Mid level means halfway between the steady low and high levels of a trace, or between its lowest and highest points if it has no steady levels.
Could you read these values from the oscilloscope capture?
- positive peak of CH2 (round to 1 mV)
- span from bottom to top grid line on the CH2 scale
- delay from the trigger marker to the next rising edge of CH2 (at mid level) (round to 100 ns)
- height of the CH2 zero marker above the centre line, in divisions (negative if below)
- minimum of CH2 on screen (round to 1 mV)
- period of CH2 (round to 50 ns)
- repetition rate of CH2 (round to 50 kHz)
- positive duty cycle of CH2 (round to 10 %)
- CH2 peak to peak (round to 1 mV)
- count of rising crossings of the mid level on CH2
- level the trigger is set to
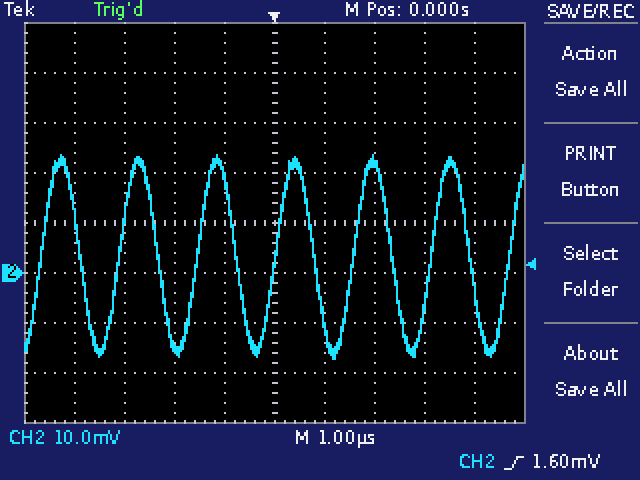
24 mV
80 mV
1.6 µs
-1.0 div
-17 mV
1.55 µs
650 kHz
50 %
41 mV
7
1.60 mV
